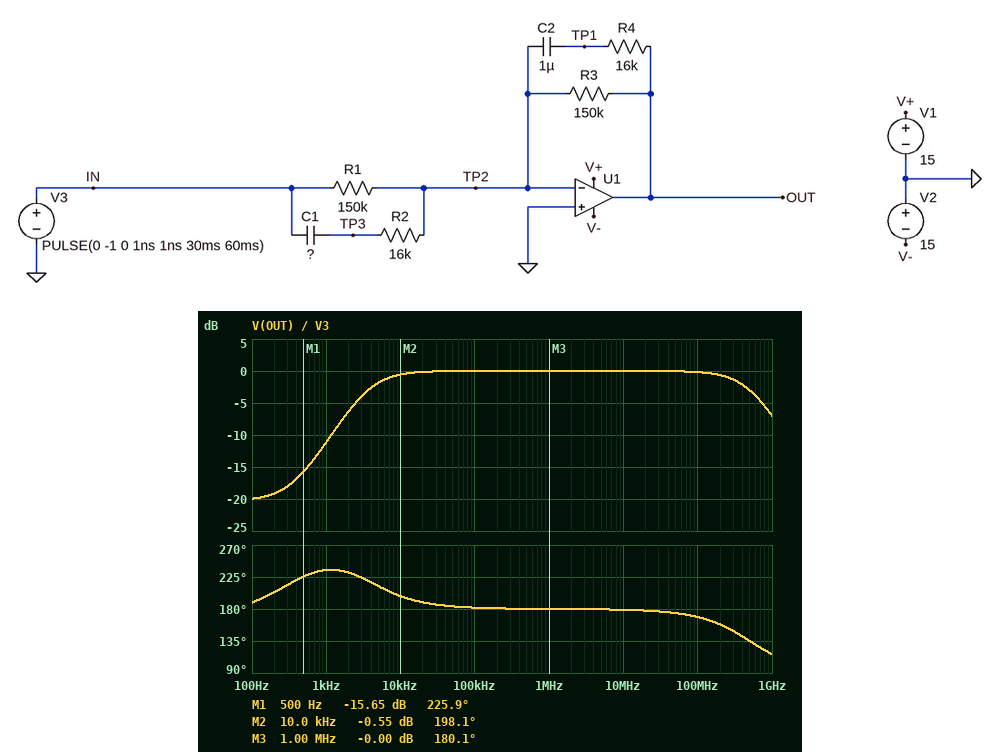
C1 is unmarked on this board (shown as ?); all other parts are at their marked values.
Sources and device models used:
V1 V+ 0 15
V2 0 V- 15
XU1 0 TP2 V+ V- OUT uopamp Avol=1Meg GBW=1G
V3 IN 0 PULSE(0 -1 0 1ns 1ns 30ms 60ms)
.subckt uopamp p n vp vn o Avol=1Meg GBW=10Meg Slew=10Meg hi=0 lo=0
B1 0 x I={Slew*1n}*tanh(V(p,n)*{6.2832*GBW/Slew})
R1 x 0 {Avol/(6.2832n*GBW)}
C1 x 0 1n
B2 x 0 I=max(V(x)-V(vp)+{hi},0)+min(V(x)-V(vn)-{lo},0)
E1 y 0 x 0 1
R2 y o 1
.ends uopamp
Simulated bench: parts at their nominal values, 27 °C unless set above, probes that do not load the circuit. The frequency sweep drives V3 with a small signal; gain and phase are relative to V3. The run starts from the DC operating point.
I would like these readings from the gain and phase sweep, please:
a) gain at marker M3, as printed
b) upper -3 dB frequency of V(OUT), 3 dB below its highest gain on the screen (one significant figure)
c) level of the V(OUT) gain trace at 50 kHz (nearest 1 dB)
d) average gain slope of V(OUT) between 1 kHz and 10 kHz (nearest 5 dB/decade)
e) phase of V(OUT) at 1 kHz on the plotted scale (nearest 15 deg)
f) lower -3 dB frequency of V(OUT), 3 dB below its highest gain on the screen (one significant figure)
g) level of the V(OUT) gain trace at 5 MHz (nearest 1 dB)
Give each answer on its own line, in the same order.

-0.00 dB
500 MHz
0 dB
10 dB/decade
240 deg
4 kHz
0 dB
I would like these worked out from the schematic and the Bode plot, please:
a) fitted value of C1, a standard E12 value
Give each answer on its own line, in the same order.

2.7 nF
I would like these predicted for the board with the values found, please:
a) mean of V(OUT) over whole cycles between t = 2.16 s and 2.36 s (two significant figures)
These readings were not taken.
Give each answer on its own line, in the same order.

500 mV
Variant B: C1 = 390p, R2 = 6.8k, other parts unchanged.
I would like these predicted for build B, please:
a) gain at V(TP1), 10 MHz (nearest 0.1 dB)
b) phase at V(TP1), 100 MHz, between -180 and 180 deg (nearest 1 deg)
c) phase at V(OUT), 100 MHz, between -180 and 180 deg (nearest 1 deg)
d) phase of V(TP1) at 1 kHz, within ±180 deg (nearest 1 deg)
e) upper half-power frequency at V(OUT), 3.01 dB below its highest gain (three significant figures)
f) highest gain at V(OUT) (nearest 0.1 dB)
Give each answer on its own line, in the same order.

-33.1 dB
72 deg
162 deg
110 deg
310 MHz
6.9 dB
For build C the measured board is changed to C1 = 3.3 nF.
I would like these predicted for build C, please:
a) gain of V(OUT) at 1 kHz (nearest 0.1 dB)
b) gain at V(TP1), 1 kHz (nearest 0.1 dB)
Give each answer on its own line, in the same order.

-9.7 dB
-49.7 dB
